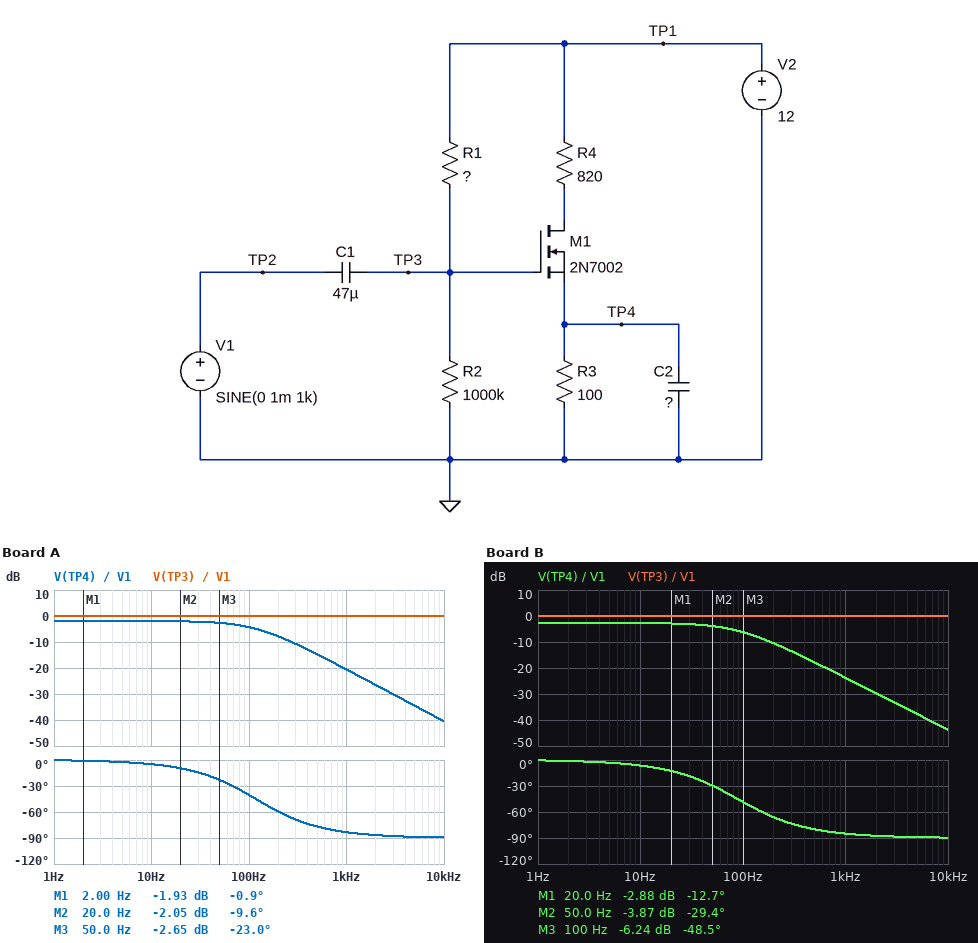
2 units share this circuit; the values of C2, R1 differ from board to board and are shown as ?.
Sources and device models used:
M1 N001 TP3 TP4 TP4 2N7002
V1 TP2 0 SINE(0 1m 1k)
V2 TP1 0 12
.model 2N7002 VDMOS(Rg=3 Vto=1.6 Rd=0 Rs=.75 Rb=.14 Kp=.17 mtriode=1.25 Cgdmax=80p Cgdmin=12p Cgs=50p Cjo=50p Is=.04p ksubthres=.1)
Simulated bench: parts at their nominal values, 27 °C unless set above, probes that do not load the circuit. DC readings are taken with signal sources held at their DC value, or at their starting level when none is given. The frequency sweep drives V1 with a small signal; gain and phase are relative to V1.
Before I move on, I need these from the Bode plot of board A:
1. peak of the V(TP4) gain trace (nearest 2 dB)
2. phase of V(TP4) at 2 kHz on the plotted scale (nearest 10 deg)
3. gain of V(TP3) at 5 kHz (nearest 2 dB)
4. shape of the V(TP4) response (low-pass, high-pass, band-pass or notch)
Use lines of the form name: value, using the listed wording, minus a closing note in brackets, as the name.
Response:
peak of the V(TP4) gain trace: -2 dB
phase of V(TP4) at 2 kHz on the plotted scale: -90 deg
gain of V(TP3) at 5 kHz: 0 dB
shape of the V(TP4) response: low-pass
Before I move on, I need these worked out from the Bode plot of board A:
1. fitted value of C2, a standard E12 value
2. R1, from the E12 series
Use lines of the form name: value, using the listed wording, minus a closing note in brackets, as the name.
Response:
fitted value of C2, a standard E12 value: 68 µF
R1, from the E12 series: 3.9 MΩ
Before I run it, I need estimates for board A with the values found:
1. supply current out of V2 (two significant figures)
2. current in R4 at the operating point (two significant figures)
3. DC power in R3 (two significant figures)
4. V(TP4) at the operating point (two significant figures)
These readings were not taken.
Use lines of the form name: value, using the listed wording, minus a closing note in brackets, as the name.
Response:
supply current out of V2: 5.9 mA
current in R4 at the operating point: 5.9 mA
DC power in R3: 3.5 mW
V(TP4) at the operating point: 590 mV
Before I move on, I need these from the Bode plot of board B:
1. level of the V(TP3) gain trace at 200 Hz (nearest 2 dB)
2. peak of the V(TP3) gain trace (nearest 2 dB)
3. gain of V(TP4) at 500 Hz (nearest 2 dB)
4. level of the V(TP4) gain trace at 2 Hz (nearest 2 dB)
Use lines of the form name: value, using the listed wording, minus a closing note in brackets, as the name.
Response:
level of the V(TP3) gain trace at 200 Hz: 0 dB
peak of the V(TP3) gain trace: 0 dB
gain of V(TP4) at 500 Hz: -18 dB
level of the V(TP4) gain trace at 2 Hz: -2 dB
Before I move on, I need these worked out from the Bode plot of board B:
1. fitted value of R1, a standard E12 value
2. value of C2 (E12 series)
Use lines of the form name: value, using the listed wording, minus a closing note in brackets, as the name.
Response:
fitted value of R1, a standard E12 value: 4.7 MΩ
value of C2: 68 µF
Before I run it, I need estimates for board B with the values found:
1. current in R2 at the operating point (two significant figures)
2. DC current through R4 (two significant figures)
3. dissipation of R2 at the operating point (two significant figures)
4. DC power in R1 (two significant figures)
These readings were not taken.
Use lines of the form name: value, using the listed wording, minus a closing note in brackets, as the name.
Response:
current in R2 at the operating point: 2.1 µA
DC current through R4: 3.2 mA
dissipation of R2 at the operating point: 4.4 µW
DC power in R1: 21 µW
